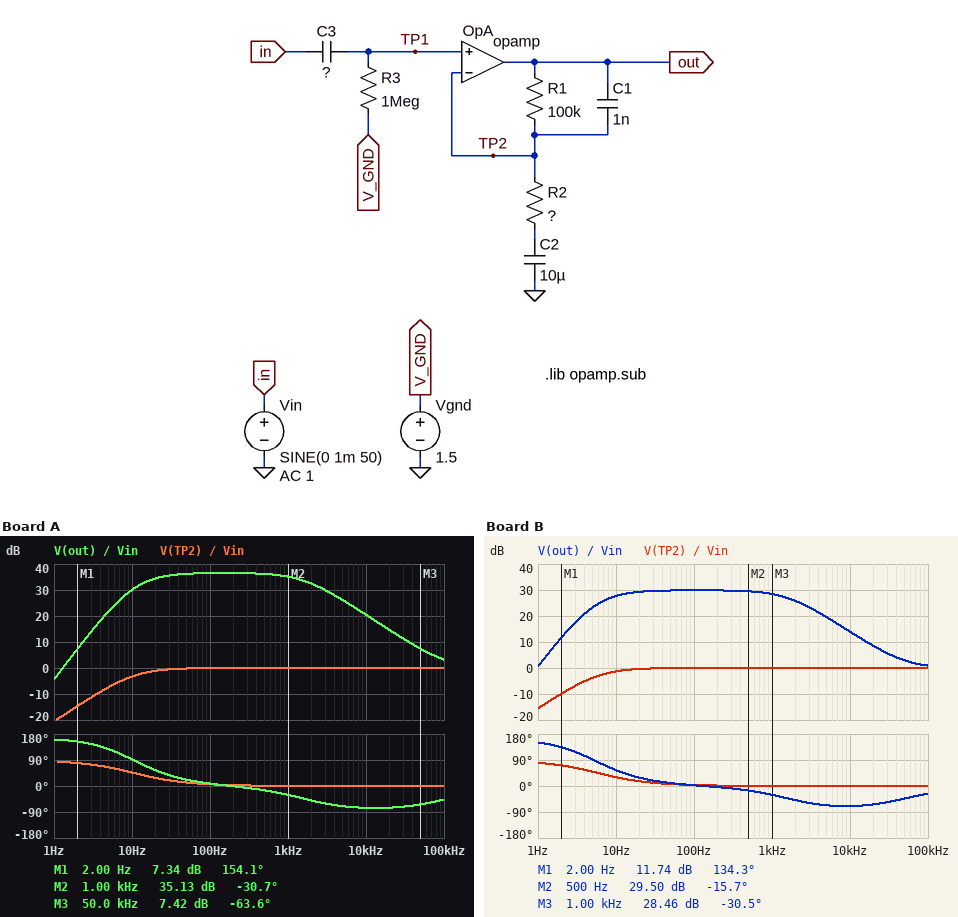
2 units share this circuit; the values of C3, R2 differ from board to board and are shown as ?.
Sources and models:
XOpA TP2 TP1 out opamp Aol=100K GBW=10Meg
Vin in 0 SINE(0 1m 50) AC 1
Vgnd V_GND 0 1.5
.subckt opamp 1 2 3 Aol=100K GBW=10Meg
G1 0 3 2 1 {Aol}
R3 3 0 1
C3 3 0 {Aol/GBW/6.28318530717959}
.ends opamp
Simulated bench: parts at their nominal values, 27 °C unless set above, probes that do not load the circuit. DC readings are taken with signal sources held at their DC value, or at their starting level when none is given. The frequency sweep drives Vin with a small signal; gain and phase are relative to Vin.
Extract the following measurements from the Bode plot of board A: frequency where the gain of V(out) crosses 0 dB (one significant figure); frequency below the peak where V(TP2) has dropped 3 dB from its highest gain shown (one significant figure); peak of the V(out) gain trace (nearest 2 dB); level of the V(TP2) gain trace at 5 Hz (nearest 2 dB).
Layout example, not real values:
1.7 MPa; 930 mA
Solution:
1 Hz; 10 Hz; 36 dB; -8 dB
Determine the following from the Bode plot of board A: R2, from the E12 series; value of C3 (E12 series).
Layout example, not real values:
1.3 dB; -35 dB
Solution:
1.5 kΩ; 15 nF
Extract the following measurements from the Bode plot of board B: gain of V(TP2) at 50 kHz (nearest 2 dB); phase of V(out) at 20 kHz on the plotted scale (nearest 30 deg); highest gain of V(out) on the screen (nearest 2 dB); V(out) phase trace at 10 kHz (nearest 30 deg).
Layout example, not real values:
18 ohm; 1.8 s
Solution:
0 dB; -60 deg; 30 dB; -60 deg
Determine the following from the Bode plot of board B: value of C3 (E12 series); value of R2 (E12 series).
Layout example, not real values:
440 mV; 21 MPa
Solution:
27 nF; 3.3 kΩ
